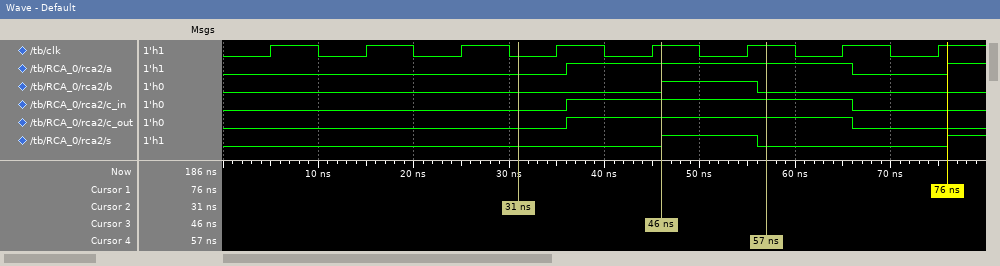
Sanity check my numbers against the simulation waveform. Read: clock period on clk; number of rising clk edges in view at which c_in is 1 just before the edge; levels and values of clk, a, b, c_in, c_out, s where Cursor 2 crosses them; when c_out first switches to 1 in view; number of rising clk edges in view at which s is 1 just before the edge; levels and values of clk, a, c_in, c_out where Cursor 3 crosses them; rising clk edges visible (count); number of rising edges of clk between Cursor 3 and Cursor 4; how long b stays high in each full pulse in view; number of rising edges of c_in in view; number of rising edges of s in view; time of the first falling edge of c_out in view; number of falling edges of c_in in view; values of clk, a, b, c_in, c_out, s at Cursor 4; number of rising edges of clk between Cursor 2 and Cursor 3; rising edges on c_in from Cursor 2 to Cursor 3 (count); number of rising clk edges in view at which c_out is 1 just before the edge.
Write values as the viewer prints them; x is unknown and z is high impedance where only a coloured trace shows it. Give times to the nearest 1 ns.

10 ns
3
clk=0, a=0, b=0, c_in=0, c_out=0, s=0
36 ns
1
clk=1, a=1, c_in=1, c_out=1
8
1
10 ns
1
2
66 ns
1
clk=1, a=1, b=0, c_in=1, c_out=1, s=0
2
1
3
